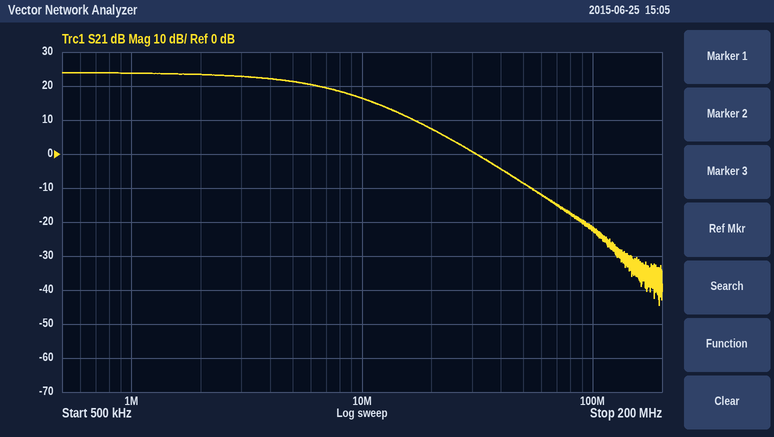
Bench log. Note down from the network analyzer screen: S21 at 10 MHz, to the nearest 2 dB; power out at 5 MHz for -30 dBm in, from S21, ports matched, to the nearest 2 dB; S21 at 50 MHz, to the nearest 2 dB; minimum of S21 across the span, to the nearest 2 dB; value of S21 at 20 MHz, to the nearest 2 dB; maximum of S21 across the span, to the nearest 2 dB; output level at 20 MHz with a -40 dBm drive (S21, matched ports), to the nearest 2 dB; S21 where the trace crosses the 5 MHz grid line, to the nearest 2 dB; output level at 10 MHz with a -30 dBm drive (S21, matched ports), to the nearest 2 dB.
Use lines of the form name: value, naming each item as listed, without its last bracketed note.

S21 at 10 MHz, to the nearest 2 dB: 16 dB
power out at 5 MHz for -30 dBm in, from S21, ports matched, to the nearest 2 dB: -8 dBm
S21 at 50 MHz, to the nearest 2 dB: -8 dB
minimum of S21 across the span, to the nearest 2 dB: -44 dB
value of S21 at 20 MHz, to the nearest 2 dB: 8 dB
maximum of S21 across the span, to the nearest 2 dB: 24 dB
output level at 20 MHz with a -40 dBm drive (S21, matched ports), to the nearest 2 dB: -32 dBm
S21 where the trace crosses the 5 MHz grid line, to the nearest 2 dB: 22 dB
output level at 10 MHz with a -30 dBm drive (S21, matched ports), to the nearest 2 dB: -14 dBm
